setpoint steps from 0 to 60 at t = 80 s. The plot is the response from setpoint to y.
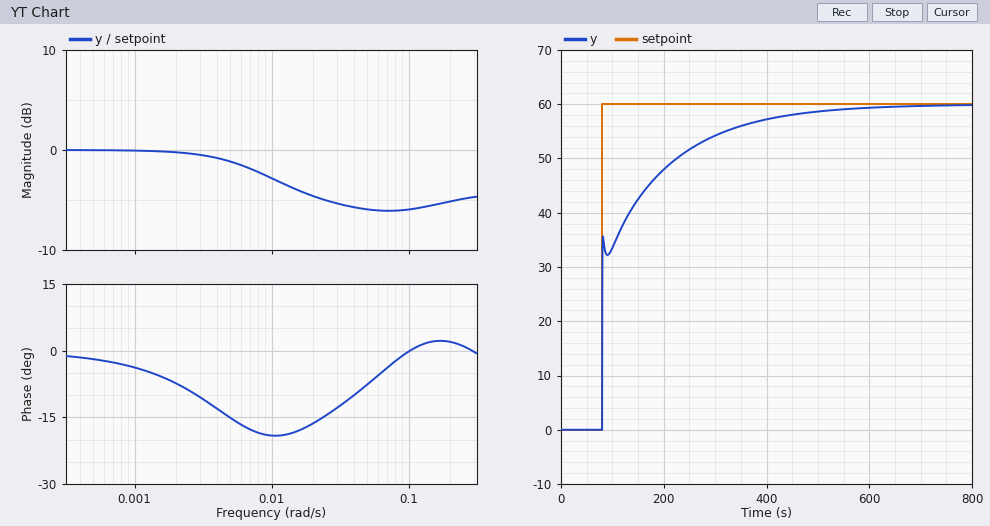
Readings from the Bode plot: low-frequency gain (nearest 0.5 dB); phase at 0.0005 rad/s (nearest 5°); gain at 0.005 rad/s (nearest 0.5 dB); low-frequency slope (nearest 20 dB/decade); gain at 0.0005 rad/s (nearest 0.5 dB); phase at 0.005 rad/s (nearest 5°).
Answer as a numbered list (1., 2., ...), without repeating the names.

1. 0.0 dB
2. 0°
3. -1.0 dB
4. 0 dB/decade
5. 0.0 dB
6. -15°
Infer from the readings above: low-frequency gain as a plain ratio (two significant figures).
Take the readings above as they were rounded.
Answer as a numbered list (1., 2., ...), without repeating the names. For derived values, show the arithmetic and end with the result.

1. 10^(0 / 20) = 1.0
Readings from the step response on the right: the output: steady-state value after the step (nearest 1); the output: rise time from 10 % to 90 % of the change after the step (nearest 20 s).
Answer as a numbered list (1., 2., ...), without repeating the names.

1. 60
2. 220 s
